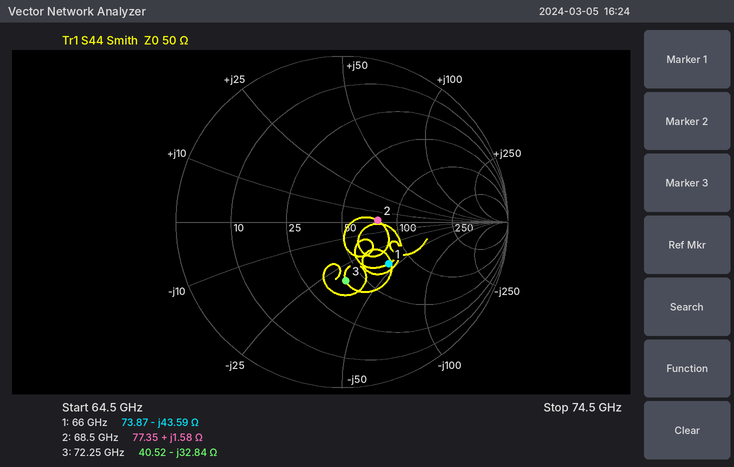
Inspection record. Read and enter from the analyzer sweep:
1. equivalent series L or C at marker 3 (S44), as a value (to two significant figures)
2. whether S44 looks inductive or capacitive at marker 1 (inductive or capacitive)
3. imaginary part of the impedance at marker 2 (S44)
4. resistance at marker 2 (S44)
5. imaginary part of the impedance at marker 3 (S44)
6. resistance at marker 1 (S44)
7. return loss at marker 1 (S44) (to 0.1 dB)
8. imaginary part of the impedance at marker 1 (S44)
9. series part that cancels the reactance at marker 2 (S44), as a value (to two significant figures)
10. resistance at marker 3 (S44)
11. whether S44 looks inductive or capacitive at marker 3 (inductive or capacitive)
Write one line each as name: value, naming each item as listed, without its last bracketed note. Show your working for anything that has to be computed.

equivalent series L or C at marker 3 (S44), as a value: C = 1/(2π × 72.25 GHz × 32.84 Ω) ≈ 67 fF
whether S44 looks inductive or capacitive at marker 1: capacitive
imaginary part of the impedance at marker 2: +1.58 Ω
resistance at marker 2: 77.35 Ω
imaginary part of the impedance at marker 3: -32.84 Ω
resistance at marker 1: 73.87 Ω
return loss at marker 1 (S44): 8.4 dB
imaginary part of the impedance at marker 1: -43.59 Ω
series part that cancels the reactance at marker 2 (S44), as a value: C = 1/(2π × 68.5 GHz × 1.58 Ω) ≈ 1.5 pF
resistance at marker 3: 40.52 Ω
whether S44 looks inductive or capacitive at marker 3: capacitive
